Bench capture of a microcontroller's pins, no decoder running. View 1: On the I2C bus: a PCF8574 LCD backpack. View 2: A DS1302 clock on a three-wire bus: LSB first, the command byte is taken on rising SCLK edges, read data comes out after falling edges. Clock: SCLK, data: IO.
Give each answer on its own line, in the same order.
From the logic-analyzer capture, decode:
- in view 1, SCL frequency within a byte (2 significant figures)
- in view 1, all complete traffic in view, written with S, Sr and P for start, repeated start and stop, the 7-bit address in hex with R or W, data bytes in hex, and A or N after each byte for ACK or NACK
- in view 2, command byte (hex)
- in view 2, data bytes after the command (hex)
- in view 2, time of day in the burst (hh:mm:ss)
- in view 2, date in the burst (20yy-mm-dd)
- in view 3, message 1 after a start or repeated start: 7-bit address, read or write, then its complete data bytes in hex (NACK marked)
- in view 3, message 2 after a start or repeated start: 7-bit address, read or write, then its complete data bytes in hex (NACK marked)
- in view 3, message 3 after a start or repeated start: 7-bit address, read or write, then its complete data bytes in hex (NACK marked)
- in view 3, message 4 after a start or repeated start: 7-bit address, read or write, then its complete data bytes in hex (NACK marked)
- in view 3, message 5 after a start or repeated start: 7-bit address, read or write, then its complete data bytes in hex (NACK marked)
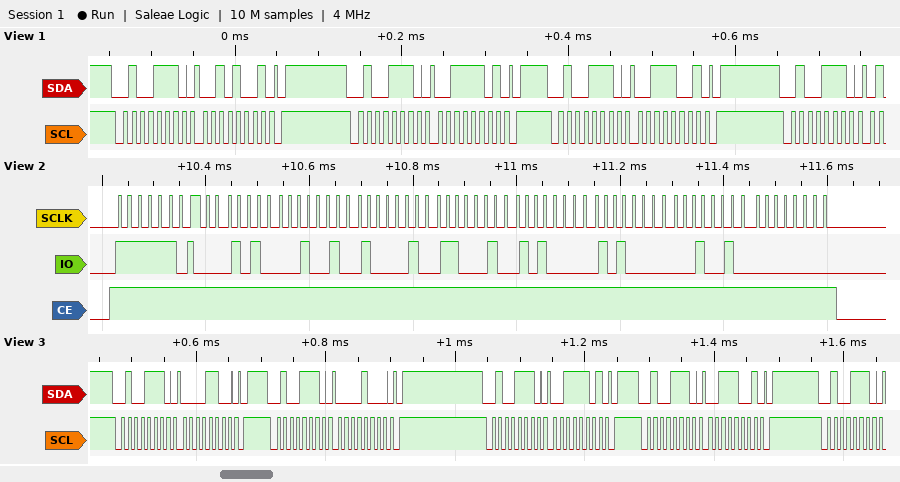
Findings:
100 kHz
S 27W A 29 A P S 27W A 3D A P S 27W A 39 A P S 27W A
0xBF
28 24 21 23 05 05 24 00
21:24:28
2024-05-23
0x27 write: 0C
0x27 write: 08
0x27 write: 3D
0x27 write: 39
0x27 write
